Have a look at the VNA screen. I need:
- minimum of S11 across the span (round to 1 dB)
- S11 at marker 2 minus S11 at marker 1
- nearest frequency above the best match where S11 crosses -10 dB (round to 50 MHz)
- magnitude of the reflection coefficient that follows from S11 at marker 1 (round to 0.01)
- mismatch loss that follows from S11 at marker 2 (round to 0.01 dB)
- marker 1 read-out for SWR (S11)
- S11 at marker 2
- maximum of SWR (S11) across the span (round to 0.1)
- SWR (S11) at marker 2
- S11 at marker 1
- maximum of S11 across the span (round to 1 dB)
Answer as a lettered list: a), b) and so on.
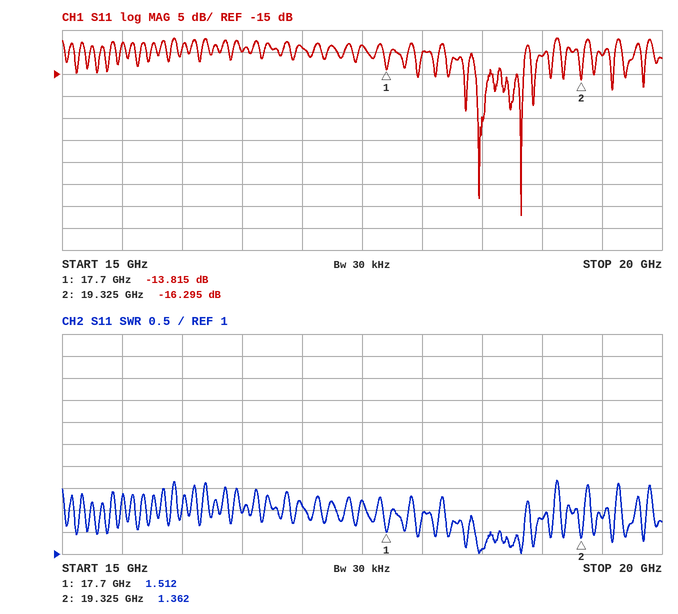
a) -47 dB
b) -2.480 dB
c) 18.85 GHz
d) 0.20
e) 0.10 dB
f) 1.512
g) -16.295 dB
h) 2.7
i) 1.362
j) -13.815 dB
k) -7 dB
